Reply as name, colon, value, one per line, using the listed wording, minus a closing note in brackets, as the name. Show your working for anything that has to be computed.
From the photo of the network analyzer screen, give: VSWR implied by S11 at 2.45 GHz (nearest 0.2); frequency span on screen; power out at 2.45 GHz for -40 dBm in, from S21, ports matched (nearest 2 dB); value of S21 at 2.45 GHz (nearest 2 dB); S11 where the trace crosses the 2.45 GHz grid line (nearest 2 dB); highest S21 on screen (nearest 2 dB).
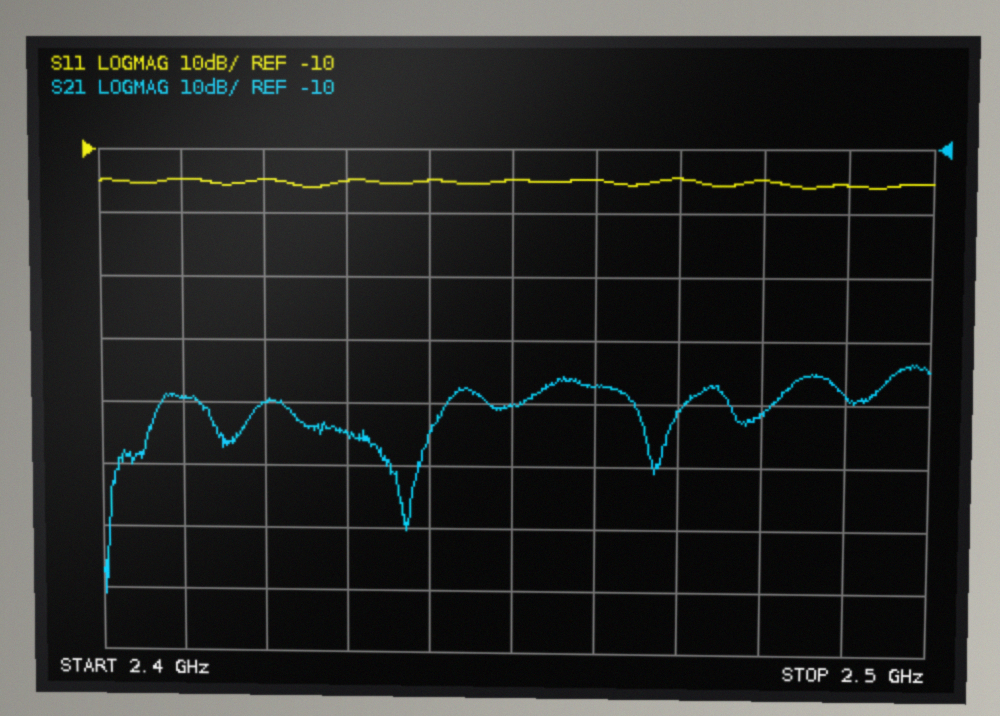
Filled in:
VSWR implied by S11 at 2.45 GHz: |Γ| = 10^(-14/20) = 0.1995; VSWR = (1 + 0.1995)/(1 − 0.1995) ≈ 1.50, so 1.4 to the nearest 0.2
frequency span on screen: 100 MHz
power out at 2.45 GHz for -40 dBm in, from S21, ports matched: -40 dBm + (-50 dB) = -90 dBm
value of S21 at 2.45 GHz: -50 dB
S11 where the trace crosses the 2.45 GHz grid line: -14 dB
highest S21 on screen: -44 dB
